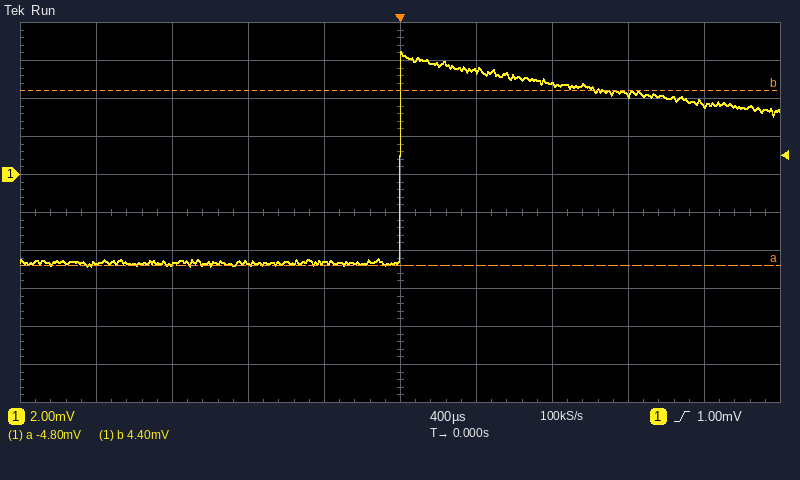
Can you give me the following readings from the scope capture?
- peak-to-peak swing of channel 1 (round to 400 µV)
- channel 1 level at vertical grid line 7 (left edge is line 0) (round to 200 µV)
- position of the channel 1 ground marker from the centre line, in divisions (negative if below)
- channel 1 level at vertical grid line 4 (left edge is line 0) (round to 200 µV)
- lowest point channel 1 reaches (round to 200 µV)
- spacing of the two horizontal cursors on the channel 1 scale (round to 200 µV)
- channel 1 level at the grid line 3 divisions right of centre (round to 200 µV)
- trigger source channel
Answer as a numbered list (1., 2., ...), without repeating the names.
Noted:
1. 11.2 mV
2. 4.8 mV
3. +1.0 div
4. -4.6 mV
5. -4.8 mV
6. 9.2 mV
7. 4.2 mV
8. channel 1
